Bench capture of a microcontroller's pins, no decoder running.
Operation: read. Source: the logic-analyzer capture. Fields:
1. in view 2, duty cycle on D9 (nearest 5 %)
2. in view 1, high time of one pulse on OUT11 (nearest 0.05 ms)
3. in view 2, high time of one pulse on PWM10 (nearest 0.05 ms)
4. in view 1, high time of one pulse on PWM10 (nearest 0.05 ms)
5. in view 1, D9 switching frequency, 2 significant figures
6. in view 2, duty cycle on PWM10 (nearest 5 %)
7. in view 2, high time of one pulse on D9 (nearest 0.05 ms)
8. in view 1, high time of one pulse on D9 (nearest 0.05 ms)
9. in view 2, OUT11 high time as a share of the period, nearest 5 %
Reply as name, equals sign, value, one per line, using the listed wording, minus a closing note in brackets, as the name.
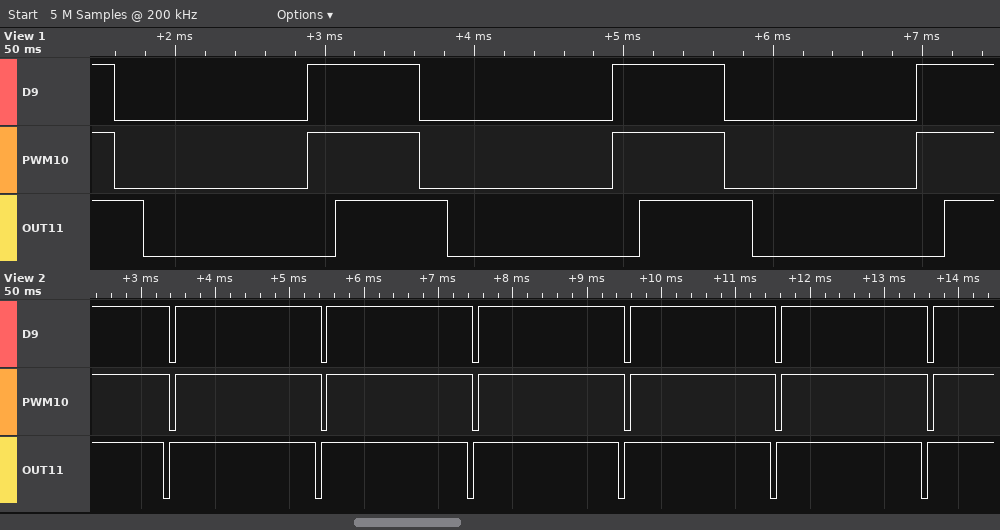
in view 2, duty cycle on D9 = 95 %
in view 1, high time of one pulse on OUT11 = 0.75 ms
in view 2, high time of one pulse on PWM10 = 1.95 ms
in view 1, high time of one pulse on PWM10 = 0.75 ms
in view 1, D9 switching frequency, 2 significant figures = 490 Hz
in view 2, duty cycle on PWM10 = 95 %
in view 2, high time of one pulse on D9 = 1.95 ms
in view 1, high time of one pulse on D9 = 0.75 ms
in view 2, OUT11 high time as a share of the period, nearest 5 % = 95 %
